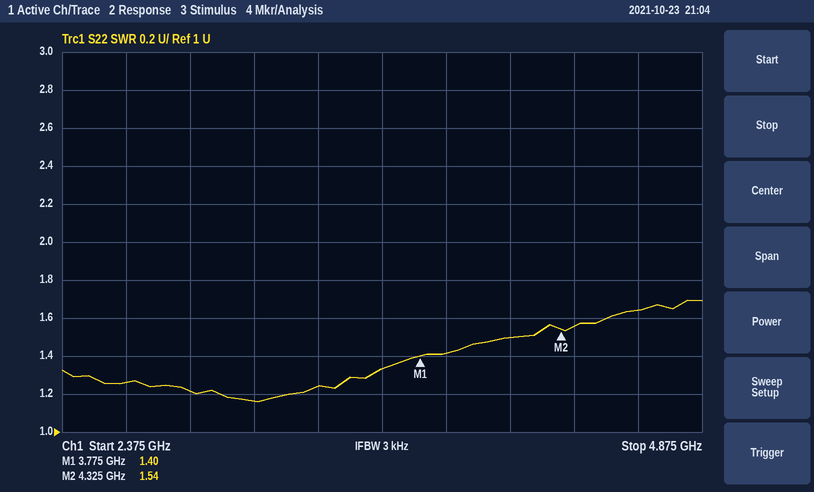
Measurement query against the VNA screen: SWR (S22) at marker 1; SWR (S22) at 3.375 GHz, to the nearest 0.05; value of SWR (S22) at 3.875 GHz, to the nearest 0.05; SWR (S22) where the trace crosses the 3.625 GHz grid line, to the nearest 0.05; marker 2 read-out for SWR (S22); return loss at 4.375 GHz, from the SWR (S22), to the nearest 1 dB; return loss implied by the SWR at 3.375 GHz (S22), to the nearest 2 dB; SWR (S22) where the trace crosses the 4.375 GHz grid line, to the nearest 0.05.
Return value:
1.40
1.25
1.40
1.35
1.54
13 dB
20 dB
1.55
